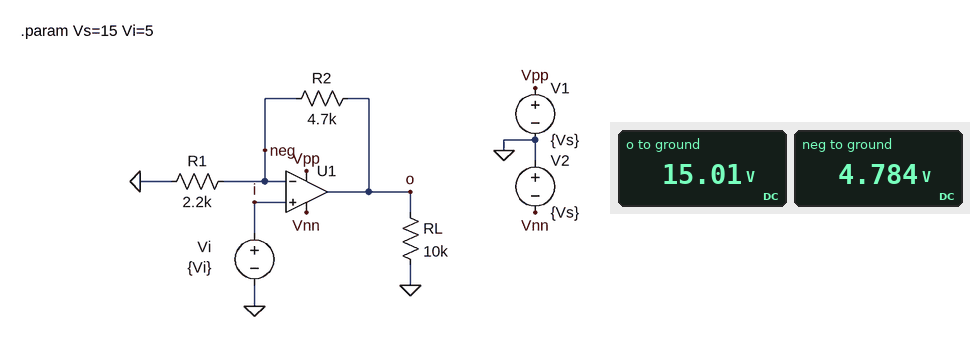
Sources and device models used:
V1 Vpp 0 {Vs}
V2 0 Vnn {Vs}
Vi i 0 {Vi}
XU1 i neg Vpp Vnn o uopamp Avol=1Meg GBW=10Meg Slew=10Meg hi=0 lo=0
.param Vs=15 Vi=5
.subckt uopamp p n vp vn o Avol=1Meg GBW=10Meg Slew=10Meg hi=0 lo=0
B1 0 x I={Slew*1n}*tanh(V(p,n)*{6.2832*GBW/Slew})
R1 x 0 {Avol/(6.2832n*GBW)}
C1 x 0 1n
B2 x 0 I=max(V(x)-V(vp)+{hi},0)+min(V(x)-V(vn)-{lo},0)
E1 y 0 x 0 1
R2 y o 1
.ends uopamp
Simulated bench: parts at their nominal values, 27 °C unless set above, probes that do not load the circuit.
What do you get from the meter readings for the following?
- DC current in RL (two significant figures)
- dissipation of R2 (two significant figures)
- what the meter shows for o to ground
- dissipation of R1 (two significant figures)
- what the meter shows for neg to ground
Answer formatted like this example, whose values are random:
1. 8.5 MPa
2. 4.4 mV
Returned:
1. 1.5 mA
2. 22 mW
3. 15.01 V
4. 10 mW
5. 4.784 V
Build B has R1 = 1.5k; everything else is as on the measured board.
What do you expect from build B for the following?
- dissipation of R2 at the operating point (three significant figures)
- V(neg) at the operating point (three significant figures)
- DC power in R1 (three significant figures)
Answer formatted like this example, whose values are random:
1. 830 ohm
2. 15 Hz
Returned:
1. 27.5 mW
2. 3.63 V
3. 8.79 mW
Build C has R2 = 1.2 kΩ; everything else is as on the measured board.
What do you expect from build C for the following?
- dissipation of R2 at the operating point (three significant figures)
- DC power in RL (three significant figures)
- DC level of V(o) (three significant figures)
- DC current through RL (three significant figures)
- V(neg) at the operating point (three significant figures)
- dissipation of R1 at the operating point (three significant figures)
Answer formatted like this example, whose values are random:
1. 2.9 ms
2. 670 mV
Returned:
1. 6.20 mW
2. 5.97 mW
3. 7.73 V
4. 773 µA
5. 5.00 V
6. 11.4 mW
